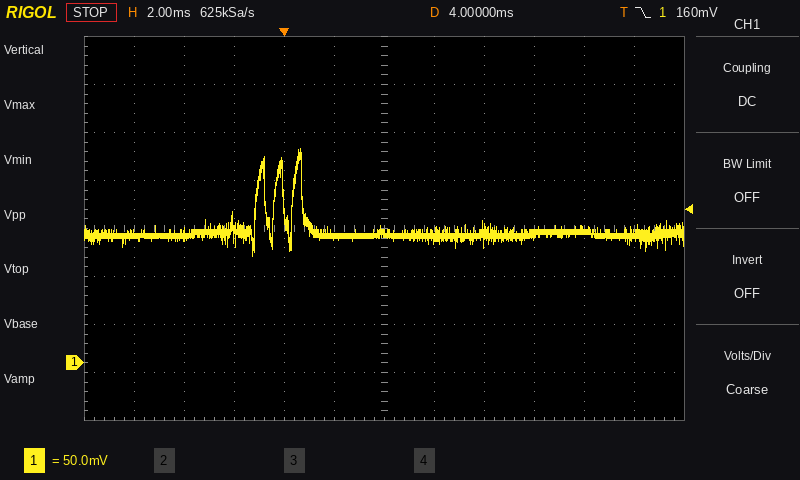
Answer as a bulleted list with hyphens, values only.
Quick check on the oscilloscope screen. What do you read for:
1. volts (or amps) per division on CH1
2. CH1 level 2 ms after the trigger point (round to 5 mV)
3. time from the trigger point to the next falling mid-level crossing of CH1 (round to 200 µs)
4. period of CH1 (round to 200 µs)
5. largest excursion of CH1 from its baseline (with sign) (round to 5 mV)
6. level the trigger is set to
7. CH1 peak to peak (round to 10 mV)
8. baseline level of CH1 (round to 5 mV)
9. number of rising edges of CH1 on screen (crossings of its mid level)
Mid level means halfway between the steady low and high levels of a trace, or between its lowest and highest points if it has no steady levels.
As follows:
- 50 mV
- 130 mV
- 800 µs
- 800 µs
- +90 mV
- 160 mV
- 110 mV
- 135 mV
- 3
